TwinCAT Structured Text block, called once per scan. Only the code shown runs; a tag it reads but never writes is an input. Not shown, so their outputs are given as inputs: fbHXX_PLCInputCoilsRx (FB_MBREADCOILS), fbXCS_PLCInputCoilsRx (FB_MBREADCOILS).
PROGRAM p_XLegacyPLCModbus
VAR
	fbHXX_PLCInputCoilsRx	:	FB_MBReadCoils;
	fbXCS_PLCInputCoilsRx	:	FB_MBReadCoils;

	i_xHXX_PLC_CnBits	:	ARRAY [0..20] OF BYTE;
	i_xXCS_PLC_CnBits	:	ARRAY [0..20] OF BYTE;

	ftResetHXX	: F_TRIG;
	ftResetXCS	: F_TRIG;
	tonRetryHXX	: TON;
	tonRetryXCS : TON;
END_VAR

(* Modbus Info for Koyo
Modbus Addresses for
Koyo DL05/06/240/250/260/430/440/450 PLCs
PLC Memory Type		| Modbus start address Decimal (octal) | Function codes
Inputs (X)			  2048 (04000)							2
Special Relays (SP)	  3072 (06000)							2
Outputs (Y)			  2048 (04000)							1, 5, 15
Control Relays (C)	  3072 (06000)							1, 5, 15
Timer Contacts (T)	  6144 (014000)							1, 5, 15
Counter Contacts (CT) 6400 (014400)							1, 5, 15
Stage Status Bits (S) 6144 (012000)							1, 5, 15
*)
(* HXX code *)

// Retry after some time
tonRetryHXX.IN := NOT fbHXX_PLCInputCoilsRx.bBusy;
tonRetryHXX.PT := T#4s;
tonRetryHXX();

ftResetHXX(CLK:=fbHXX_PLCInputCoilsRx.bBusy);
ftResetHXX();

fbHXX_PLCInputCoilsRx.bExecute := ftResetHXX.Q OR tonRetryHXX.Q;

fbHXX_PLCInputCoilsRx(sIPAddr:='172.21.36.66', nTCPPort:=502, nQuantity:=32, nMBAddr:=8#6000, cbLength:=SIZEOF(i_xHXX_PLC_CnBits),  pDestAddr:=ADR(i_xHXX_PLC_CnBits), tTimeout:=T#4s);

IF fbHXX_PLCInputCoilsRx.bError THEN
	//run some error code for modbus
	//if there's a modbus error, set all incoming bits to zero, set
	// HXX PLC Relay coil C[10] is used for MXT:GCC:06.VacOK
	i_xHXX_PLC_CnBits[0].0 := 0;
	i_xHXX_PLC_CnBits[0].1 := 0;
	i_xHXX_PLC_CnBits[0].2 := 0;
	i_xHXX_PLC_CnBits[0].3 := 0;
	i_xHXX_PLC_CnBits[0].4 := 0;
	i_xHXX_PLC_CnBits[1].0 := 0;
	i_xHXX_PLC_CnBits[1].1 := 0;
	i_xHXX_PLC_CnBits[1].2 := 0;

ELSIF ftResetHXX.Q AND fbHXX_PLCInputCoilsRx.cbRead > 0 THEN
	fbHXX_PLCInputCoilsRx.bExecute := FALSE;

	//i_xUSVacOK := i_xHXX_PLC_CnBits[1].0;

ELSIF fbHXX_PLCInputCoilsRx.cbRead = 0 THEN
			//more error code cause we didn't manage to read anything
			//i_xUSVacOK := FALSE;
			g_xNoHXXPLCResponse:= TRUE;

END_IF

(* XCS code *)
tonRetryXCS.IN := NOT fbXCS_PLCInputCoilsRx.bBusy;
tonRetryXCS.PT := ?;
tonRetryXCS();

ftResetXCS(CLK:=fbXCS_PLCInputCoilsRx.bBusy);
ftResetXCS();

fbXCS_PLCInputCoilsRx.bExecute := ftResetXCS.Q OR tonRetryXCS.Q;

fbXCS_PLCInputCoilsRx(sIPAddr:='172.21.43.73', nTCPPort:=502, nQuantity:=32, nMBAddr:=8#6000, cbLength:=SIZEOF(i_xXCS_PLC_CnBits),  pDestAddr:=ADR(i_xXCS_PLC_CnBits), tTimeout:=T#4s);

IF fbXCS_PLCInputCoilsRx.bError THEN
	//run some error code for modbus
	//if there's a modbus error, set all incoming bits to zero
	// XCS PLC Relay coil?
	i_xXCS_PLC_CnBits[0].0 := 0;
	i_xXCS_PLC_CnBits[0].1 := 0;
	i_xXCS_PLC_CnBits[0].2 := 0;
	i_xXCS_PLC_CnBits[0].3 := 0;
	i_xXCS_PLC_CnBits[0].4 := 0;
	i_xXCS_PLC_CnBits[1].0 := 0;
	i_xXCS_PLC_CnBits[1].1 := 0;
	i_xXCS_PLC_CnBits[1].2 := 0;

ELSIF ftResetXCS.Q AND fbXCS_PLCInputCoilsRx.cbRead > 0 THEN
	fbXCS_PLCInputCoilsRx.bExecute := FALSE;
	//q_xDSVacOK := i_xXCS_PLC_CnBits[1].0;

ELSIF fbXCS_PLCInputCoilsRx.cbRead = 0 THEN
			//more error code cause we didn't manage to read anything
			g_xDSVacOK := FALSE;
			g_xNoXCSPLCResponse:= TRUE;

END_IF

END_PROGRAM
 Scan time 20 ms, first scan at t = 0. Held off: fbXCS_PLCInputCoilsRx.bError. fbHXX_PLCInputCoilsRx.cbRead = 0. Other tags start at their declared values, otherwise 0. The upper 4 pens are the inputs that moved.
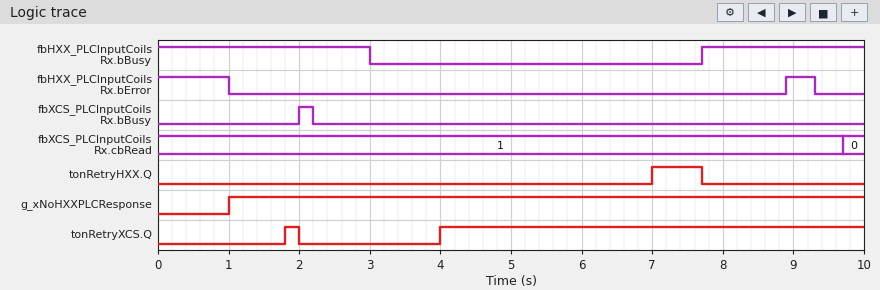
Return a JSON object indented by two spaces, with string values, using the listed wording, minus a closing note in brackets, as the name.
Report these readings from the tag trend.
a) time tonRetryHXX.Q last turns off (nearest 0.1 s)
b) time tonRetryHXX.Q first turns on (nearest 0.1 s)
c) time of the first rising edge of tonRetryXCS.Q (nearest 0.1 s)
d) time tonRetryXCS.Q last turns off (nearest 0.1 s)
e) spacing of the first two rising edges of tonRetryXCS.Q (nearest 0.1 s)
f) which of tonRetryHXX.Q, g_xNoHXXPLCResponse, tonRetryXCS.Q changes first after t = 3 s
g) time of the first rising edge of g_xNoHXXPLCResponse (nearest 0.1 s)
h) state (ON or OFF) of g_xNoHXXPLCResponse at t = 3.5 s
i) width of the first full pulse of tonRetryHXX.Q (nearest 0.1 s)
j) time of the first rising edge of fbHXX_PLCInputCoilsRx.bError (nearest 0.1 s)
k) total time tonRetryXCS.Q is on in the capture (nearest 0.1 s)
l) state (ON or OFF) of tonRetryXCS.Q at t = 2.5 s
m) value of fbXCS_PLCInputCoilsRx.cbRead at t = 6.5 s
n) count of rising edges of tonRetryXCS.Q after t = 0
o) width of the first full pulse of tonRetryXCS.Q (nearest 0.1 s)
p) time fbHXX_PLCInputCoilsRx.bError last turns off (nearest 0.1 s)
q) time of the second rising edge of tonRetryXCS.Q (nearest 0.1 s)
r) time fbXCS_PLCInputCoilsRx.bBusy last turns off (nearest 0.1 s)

{
  "time tonRetryHXX.Q last turns off": "7.7 s",
  "time tonRetryHXX.Q first turns on": "7.0 s",
  "time of the first rising edge of tonRetryXCS.Q": "1.8 s",
  "time tonRetryXCS.Q last turns off": "2.0 s",
  "spacing of the first two rising edges of tonRetryXCS.Q": "2.2 s",
  "which of tonRetryHXX.Q, g_xNoHXXPLCResponse, tonRetryXCS.Q changes first after t = 3 s": "tonRetryXCS.Q",
  "time of the first rising edge of g_xNoHXXPLCResponse": "1.0 s",
  "state (ON or OFF) of g_xNoHXXPLCResponse at t = 3.5 s": "ON",
  "width of the first full pulse of tonRetryHXX.Q": "0.7 s",
  "time of the first rising edge of fbHXX_PLCInputCoilsRx.bError": "8.9 s",
  "total time tonRetryXCS.Q is on in the capture": "6.2 s",
  "state (ON or OFF) of tonRetryXCS.Q at t = 2.5 s": "OFF",
  "value of fbXCS_PLCInputCoilsRx.cbRead at t = 6.5 s": "1",
  "count of rising edges of tonRetryXCS.Q after t = 0": "2",
  "width of the first full pulse of tonRetryXCS.Q": "0.2 s",
  "time fbHXX_PLCInputCoilsRx.bError last turns off": "9.3 s",
  "time of the second rising edge of tonRetryXCS.Q": "4.0 s",
  "time fbXCS_PLCInputCoilsRx.bBusy last turns off": "2.2 s"
}
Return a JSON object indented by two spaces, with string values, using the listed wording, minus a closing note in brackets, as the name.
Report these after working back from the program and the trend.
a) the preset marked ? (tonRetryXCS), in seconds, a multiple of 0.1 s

{
  "the preset marked ? (tonRetryXCS), in seconds, a multiple of 0.1 s": "1.8 s"
}
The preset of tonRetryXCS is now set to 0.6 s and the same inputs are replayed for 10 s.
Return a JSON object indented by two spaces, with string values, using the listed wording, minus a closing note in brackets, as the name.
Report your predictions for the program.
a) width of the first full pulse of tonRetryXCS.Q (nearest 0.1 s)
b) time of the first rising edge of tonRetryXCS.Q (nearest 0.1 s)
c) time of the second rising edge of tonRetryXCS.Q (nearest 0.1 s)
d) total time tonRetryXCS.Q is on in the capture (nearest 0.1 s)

{
  "width of the first full pulse of tonRetryXCS.Q": "1.4 s",
  "time of the first rising edge of tonRetryXCS.Q": "0.6 s",
  "time of the second rising edge of tonRetryXCS.Q": "2.8 s",
  "total time tonRetryXCS.Q is on in the capture": "8.6 s"
}
